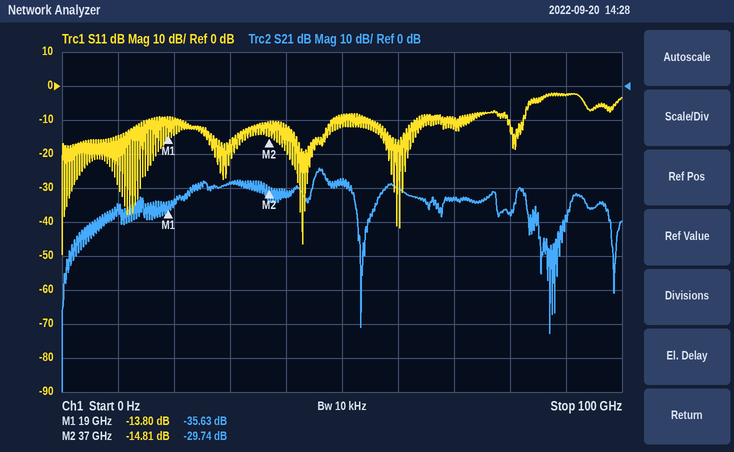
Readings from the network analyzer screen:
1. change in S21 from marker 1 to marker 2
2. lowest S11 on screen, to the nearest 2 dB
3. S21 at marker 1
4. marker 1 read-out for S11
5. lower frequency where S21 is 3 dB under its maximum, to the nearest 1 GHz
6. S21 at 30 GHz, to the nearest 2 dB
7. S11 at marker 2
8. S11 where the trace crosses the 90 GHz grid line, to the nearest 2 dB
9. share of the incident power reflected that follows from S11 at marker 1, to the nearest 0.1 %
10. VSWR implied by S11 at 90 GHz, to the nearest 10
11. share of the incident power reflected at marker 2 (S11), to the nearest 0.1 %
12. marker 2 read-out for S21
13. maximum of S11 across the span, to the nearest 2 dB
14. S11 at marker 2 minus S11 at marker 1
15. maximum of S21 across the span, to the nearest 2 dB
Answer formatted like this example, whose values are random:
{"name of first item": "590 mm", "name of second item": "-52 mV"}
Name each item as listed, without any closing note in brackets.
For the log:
{"change in S21 from marker 1 to marker 2": "5.89 dB", "lowest S11 on screen, to the nearest 2 dB": "-50 dB", "S21 at marker 1": "-35.63 dB", "marker 1 read-out for S11": "-13.80 dB", "lower frequency where S21 is 3 dB under its maximum, to the nearest 1 GHz": "45 GHz", "S21 at 30 GHz, to the nearest 2 dB": "-28 dB", "S11 at marker 2": "-14.81 dB", "S11 where the trace crosses the 90 GHz grid line, to the nearest 2 dB": "-2 dB", "share of the incident power reflected that follows from S11 at marker 1, to the nearest 0.1 %": "4.2 %", "VSWR implied by S11 at 90 GHz, to the nearest 10": "10", "share of the incident power reflected at marker 2 (S11), to the nearest 0.1 %": "3.3 %", "marker 2 read-out for S21": "-29.74 dB", "maximum of S11 across the span, to the nearest 2 dB": "-2 dB", "S11 at marker 2 minus S11 at marker 1": "-1.01 dB", "maximum of S21 across the span, to the nearest 2 dB": "-24 dB"}
